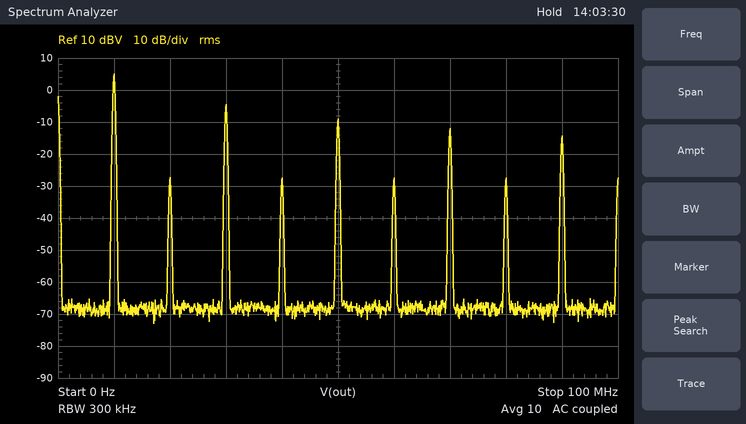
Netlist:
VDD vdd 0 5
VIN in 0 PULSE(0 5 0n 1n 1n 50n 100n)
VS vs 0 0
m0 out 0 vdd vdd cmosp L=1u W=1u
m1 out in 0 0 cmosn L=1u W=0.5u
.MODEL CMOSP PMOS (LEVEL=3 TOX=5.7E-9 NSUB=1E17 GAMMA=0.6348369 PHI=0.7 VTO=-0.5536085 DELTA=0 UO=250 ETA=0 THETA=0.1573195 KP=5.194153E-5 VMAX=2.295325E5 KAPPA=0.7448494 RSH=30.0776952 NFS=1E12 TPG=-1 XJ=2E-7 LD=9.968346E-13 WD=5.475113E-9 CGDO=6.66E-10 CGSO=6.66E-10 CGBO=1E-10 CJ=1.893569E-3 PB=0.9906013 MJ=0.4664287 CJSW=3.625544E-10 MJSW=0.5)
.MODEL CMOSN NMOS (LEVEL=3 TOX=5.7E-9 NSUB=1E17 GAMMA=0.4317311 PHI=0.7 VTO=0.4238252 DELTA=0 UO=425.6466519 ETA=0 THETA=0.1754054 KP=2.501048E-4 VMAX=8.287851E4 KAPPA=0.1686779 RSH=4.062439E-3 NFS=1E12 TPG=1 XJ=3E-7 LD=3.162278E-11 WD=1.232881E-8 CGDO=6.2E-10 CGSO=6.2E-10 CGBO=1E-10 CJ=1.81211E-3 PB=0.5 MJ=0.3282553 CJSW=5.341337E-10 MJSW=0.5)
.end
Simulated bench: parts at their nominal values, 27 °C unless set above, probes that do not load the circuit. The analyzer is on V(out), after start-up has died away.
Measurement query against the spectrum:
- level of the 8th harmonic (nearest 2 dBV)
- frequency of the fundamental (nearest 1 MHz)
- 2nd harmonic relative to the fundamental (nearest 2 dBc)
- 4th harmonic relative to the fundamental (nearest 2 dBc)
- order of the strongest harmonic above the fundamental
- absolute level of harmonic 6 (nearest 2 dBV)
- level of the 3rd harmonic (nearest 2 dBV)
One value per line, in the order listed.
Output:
-28 dBV
10 MHz
-32 dBc
-32 dBc
3
-28 dBV
-4 dBV
